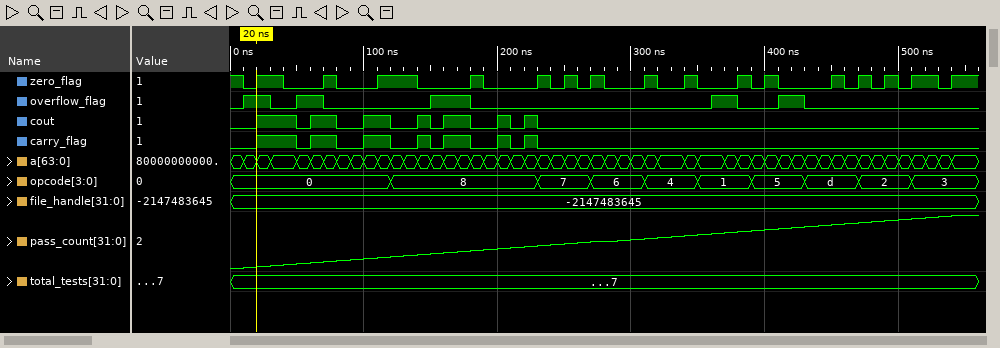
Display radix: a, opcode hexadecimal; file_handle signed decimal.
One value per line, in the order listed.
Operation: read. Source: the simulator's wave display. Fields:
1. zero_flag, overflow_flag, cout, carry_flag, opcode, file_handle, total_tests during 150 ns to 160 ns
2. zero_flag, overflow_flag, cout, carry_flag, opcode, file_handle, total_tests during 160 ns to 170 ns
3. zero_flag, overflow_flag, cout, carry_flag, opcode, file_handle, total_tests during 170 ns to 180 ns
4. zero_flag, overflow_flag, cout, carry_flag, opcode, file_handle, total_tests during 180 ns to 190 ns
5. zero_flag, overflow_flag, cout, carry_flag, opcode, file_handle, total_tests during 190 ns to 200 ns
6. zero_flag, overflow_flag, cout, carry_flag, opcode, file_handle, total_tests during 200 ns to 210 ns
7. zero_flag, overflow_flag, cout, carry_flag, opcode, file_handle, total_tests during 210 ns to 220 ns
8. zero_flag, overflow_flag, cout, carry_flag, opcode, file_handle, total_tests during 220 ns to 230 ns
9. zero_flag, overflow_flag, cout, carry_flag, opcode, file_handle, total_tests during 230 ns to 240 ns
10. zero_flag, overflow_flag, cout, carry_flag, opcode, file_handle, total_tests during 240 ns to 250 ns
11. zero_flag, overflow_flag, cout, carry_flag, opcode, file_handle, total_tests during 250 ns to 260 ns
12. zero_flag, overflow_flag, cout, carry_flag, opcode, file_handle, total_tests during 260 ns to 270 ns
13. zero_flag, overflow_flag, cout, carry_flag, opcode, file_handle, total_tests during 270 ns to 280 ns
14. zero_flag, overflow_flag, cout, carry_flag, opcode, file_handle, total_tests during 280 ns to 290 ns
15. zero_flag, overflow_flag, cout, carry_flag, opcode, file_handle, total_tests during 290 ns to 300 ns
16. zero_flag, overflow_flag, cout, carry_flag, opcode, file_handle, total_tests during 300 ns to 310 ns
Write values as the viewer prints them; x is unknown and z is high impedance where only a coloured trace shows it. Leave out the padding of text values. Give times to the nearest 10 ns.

zero_flag=0, overflow_flag=1, cout=0, carry_flag=0, opcode=8, file_handle=-2147483645, total_tests=7
zero_flag=0, overflow_flag=1, cout=1, carry_flag=1, opcode=8, file_handle=-2147483645, total_tests=7
zero_flag=0, overflow_flag=1, cout=1, carry_flag=1, opcode=8, file_handle=-2147483645, total_tests=7
zero_flag=1, overflow_flag=0, cout=0, carry_flag=0, opcode=8, file_handle=-2147483645, total_tests=7
zero_flag=0, overflow_flag=0, cout=0, carry_flag=0, opcode=8, file_handle=-2147483645, total_tests=7
zero_flag=0, overflow_flag=0, cout=1, carry_flag=1, opcode=8, file_handle=-2147483645, total_tests=7
zero_flag=0, overflow_flag=0, cout=0, carry_flag=0, opcode=8, file_handle=-2147483645, total_tests=7
zero_flag=0, overflow_flag=0, cout=1, carry_flag=1, opcode=8, file_handle=-2147483645, total_tests=7
zero_flag=1, overflow_flag=0, cout=0, carry_flag=0, opcode=7, file_handle=-2147483645, total_tests=7
zero_flag=0, overflow_flag=0, cout=0, carry_flag=0, opcode=7, file_handle=-2147483645, total_tests=7
zero_flag=1, overflow_flag=0, cout=0, carry_flag=0, opcode=7, file_handle=-2147483645, total_tests=7
zero_flag=0, overflow_flag=0, cout=0, carry_flag=0, opcode=7, file_handle=-2147483645, total_tests=7
zero_flag=1, overflow_flag=0, cout=0, carry_flag=0, opcode=6, file_handle=-2147483645, total_tests=7
zero_flag=0, overflow_flag=0, cout=0, carry_flag=0, opcode=6, file_handle=-2147483645, total_tests=7
zero_flag=0, overflow_flag=0, cout=0, carry_flag=0, opcode=6, file_handle=-2147483645, total_tests=7
zero_flag=0, overflow_flag=0, cout=0, carry_flag=0, opcode=6, file_handle=-2147483645, total_tests=7
